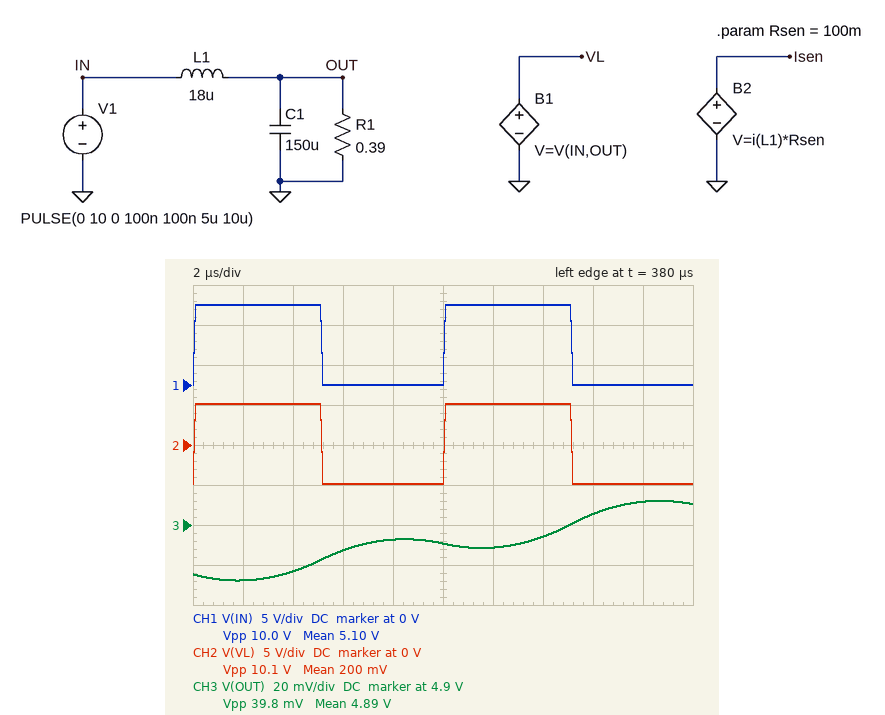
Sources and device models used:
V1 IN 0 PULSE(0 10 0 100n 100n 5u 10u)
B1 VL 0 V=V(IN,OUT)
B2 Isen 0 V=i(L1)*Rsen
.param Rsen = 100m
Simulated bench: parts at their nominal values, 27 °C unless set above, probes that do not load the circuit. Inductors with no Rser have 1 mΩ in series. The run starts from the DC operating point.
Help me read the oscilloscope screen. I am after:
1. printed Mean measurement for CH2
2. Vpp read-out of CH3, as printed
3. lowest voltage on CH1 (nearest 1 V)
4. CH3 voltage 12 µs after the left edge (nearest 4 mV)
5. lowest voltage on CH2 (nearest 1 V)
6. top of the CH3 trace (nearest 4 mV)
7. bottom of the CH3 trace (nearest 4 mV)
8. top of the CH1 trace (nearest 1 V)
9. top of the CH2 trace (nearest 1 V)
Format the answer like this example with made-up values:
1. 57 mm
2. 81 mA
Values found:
1. 200 mV
2. 39.8 mV
3. 0 V
4. 4.888 V
5. -5 V
6. 4.912 V
7. 4.872 V
8. 10 V
9. 5 V
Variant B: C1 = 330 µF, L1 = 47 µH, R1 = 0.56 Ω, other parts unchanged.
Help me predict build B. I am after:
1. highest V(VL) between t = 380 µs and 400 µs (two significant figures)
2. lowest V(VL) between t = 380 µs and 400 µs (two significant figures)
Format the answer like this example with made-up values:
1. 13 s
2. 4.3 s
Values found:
1. 3.3 V
2. -6.7 V
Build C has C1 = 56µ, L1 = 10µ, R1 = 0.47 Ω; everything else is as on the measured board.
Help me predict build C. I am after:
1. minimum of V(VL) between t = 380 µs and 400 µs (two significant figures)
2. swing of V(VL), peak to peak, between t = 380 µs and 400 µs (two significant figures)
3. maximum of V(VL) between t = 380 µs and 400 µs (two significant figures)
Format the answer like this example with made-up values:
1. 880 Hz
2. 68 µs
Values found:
1. -5.1 V
2. 10 V
3. 4.9 V
